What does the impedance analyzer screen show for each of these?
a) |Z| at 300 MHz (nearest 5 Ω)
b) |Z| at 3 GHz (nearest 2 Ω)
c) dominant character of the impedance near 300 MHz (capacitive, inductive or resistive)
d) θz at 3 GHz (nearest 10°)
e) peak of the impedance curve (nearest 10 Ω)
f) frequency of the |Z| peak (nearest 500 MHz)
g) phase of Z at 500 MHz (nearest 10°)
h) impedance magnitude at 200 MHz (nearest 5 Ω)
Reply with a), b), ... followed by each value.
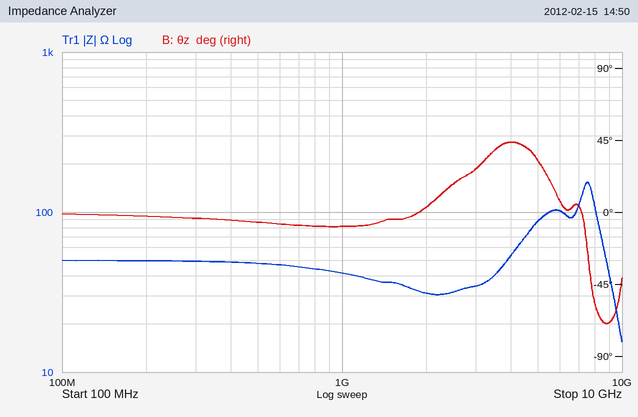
a) 50 Ω
b) 34 Ω
c) resistive
d) 30°
e) 150 Ω
f) 7.5 GHz
g) -10°
h) 50 Ω
